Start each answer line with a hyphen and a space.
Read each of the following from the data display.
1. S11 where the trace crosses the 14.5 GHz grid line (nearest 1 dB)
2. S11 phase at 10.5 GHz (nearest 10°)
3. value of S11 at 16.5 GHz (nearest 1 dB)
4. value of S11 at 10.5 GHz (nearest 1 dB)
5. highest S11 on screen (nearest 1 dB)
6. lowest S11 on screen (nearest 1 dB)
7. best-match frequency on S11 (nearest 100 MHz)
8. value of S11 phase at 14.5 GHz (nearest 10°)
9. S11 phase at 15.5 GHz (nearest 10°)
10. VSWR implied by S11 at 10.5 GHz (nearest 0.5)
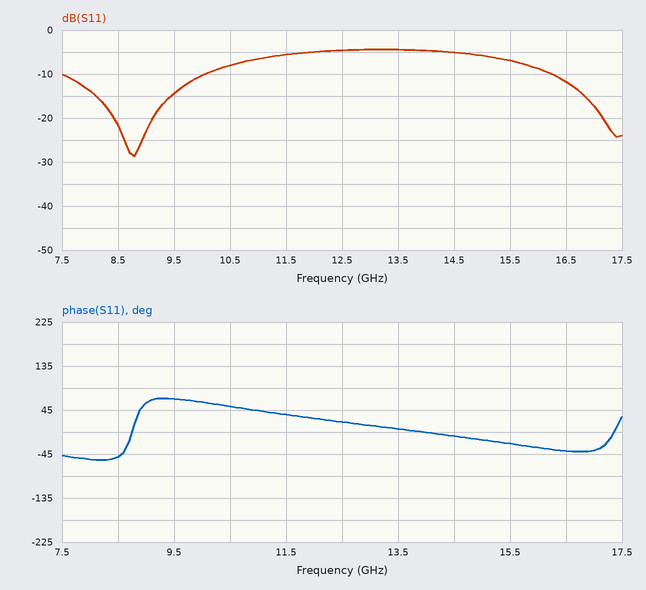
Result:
- -5 dB
- 50°
- -12 dB
- -8 dB
- -4 dB
- -29 dB
- 8.8 GHz
- -10°
- -20°
- 2.5
